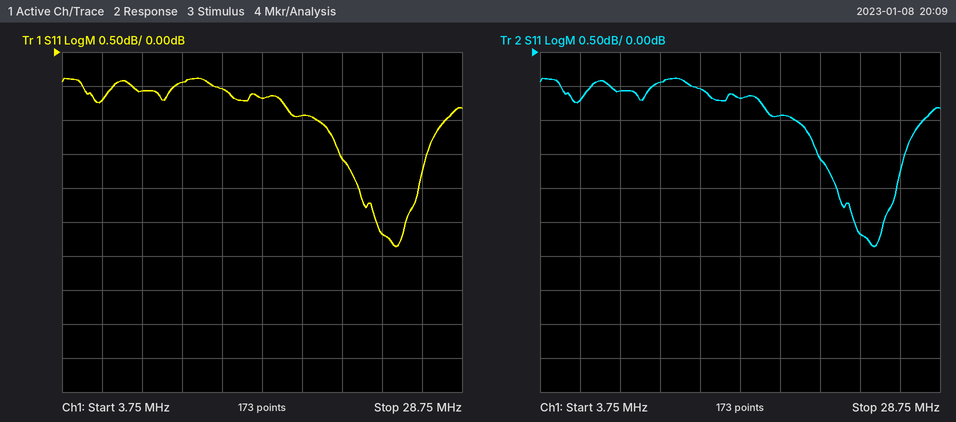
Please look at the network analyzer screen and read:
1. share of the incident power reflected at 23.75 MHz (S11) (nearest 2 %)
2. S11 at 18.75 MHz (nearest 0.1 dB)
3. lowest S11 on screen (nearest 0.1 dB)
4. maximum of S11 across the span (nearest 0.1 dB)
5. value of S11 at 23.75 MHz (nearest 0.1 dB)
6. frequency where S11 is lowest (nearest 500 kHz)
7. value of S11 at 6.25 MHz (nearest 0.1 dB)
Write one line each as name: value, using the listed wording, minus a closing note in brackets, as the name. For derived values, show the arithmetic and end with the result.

share of the incident power reflected at 23.75 MHz (S11): 10^(-2.7/10) ≈ 54 %
S11 at 18.75 MHz: -0.9 dB
lowest S11 on screen: -2.9 dB
maximum of S11 across the span: -0.4 dB
value of S11 at 23.75 MHz: -2.7 dB
frequency where S11 is lowest: 24.5 MHz
value of S11 at 6.25 MHz: -0.7 dB
